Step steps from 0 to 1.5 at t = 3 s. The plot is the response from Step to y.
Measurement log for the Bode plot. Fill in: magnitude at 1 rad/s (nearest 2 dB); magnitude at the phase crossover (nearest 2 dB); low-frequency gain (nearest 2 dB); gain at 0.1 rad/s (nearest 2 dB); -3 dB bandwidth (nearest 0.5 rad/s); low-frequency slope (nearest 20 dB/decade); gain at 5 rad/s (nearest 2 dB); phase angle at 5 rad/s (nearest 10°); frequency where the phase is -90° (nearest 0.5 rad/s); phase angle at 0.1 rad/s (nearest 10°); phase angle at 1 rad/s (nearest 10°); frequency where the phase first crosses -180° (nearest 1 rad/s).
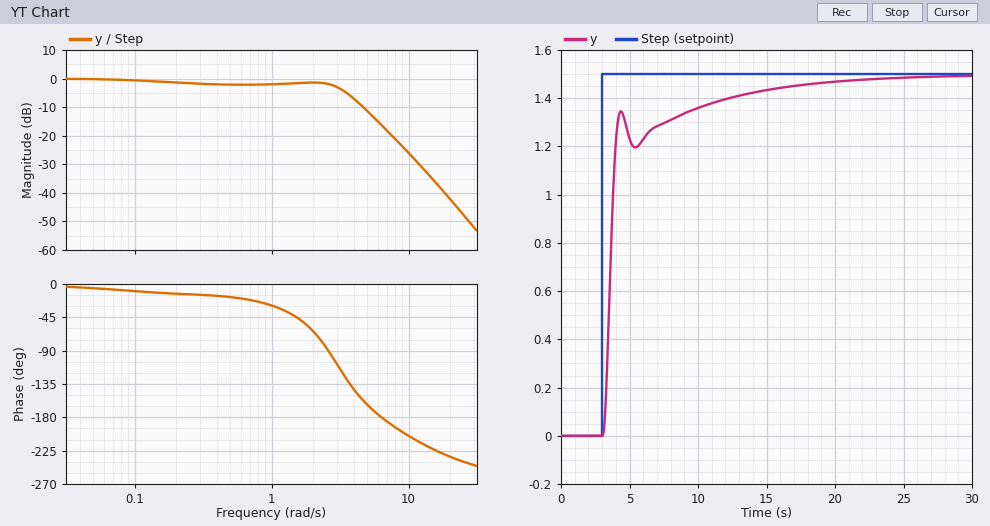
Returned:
-2 dB
-16 dB
0 dB
0 dB
3.0 rad/s
0 dB/decade
-12 dB
-160°
2.5 rad/s
-10°
-30°
6 rad/s
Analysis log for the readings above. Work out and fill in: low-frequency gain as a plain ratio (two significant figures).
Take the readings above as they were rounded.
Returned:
1.0
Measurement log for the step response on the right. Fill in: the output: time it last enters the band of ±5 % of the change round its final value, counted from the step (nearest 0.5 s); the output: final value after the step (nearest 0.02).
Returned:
11.0 s
1.50
